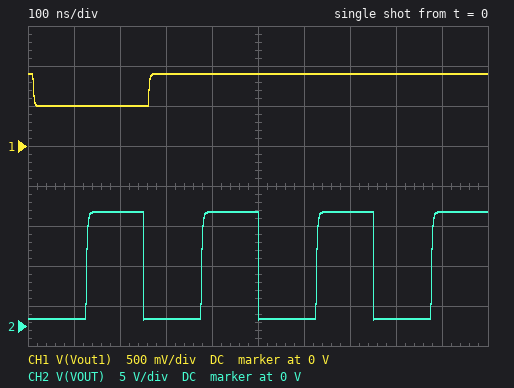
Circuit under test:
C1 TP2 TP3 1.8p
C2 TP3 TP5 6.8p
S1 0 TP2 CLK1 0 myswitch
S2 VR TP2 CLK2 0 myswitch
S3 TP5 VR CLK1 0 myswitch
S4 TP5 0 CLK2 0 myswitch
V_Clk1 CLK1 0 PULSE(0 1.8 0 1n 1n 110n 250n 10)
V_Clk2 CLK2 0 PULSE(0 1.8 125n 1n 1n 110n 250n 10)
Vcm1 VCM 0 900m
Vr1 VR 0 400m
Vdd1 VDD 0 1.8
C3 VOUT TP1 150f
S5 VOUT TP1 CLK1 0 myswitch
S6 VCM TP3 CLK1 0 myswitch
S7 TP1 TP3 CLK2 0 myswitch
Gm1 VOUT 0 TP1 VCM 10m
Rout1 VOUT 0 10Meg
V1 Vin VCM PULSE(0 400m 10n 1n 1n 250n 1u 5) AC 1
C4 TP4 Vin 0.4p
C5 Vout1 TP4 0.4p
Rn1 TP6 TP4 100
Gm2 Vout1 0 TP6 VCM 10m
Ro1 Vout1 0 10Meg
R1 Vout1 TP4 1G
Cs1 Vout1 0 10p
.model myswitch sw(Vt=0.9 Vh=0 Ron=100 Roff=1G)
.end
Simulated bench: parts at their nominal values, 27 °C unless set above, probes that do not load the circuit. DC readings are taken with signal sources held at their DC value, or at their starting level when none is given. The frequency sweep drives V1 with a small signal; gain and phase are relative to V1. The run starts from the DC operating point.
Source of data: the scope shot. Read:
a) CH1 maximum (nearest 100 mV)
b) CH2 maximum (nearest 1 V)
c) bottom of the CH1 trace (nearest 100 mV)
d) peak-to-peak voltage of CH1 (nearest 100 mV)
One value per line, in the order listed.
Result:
900 mV
14 V
500 mV
400 mV
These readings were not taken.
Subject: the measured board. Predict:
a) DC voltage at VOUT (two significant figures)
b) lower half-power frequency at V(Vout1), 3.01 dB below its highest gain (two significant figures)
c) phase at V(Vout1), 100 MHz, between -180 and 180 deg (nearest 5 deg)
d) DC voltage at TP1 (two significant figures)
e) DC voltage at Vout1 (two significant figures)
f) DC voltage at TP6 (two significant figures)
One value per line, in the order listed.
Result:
900 mV
400 Hz
125 deg
900 mV
900 mV
900 mV
